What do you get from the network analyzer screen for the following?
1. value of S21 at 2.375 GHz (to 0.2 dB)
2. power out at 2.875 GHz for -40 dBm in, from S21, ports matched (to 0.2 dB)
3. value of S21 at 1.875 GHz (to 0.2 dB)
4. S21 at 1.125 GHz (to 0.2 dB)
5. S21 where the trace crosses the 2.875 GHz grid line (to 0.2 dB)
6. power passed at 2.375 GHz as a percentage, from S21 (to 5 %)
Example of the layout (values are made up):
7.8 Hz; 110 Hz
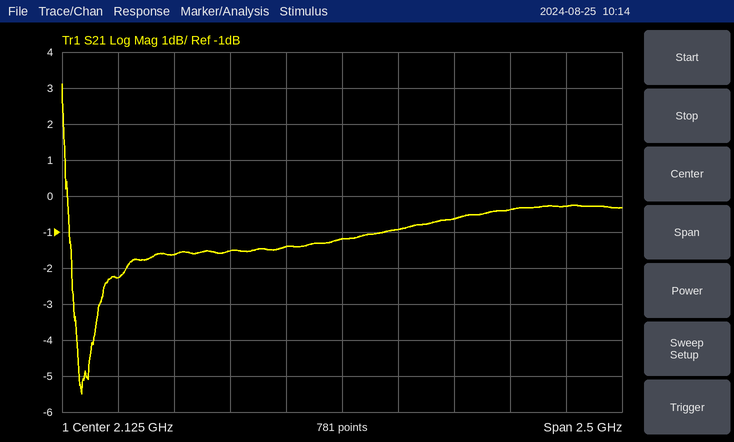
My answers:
-1.0 dB; -40.4 dBm; -1.4 dB; -2.2 dB; -0.4 dB; 80 %
